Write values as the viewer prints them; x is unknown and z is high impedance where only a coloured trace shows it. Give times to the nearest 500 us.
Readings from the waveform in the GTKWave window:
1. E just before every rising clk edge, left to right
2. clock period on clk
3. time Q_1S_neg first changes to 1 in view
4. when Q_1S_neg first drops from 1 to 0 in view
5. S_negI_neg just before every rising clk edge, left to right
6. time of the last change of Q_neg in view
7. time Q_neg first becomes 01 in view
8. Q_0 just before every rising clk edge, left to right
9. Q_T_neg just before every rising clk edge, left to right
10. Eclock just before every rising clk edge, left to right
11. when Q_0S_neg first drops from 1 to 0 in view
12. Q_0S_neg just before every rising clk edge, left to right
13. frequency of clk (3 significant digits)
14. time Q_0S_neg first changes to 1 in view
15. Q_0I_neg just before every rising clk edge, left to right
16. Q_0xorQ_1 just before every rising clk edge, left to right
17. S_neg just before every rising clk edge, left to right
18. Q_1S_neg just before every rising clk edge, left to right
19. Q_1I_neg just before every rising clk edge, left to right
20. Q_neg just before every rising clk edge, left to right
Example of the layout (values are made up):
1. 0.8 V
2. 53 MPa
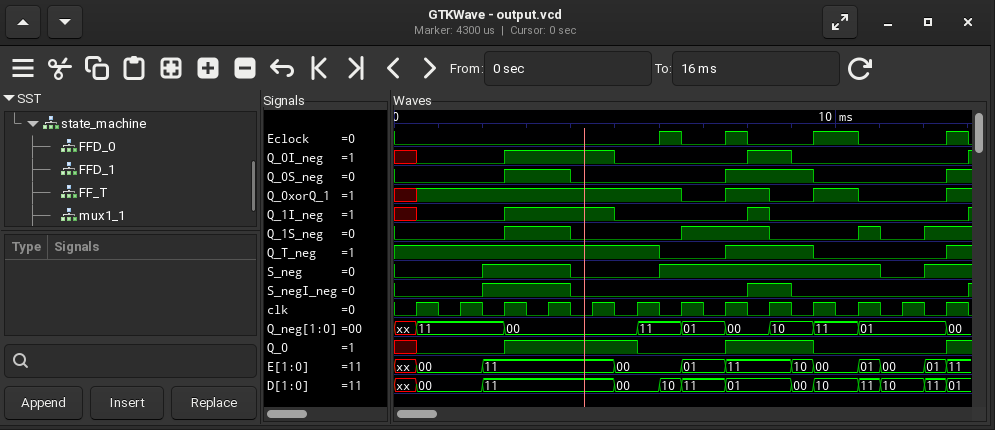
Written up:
1. xx, 00, 11, 11, 11, 00, 00, 01, 11, 10, 00, 00, 01
2. 1000 us
3. 2500 us
4. 4000 us
5. 0 0 1 1 0 0 0 0 1 0 0 0 0
6. 12500 us
7. 6500 us
8. x 0 0 1 1 1 0 0 1 1 0 0 0
9. 1 1 1 1 1 1 0 0 1 1 0 0 0
10. 0 0 0 0 0 0 1 0 0 0 1 0 0
11. 4000 us
12. 0 0 0 1 0 0 0 0 1 1 0 0 0
13. 1.00 kHz
14. 2500 us
15. x 0 0 1 1 0 0 0 1 0 0 0 0
16. x 1 1 1 1 1 1 0 1 0 1 0 0
17. 0 0 1 1 0 0 1 1 1 1 1 0 1
18. 0 0 0 1 0 0 0 1 1 0 0 0 1
19. x 0 0 1 1 0 0 0 1 0 0 0 0
20. xx, 11, 11, 00, 00, 00, 11, 01, 00, 10, 11, 01, 01
